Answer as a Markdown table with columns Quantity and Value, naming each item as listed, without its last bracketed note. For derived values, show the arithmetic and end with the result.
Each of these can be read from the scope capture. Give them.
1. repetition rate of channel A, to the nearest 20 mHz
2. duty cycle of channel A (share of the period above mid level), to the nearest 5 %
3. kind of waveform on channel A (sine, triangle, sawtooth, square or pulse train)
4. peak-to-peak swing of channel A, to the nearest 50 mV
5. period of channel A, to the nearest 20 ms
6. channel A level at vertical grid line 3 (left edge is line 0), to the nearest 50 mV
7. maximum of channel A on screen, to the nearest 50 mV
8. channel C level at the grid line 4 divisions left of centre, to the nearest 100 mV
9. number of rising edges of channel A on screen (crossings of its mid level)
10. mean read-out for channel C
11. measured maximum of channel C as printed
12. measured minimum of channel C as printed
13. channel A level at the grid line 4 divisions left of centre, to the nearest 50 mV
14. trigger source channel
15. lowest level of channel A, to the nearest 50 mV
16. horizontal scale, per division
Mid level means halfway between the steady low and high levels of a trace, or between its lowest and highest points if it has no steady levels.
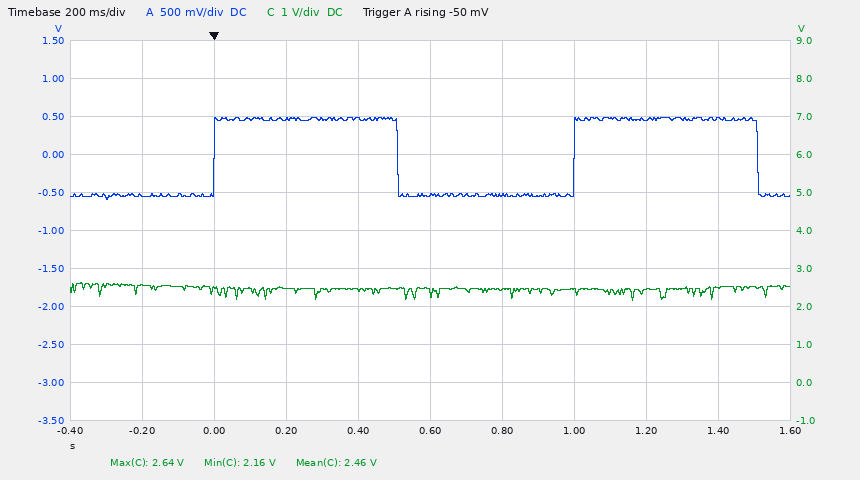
| Quantity | Value |
|---|---|
| repetition rate of channel A, to the nearest 20 mHz | 1 / 1.00 s ≈ 1.00 Hz |
| duty cycle of channel A (share of the period above mid level), to the nearest 5 % | 50 % |
| kind of waveform on channel A | square |
| peak-to-peak swing of channel A, to the nearest 50 mV | 500 mV − (-600 mV) = 1.10 V |
| period of channel A, to the nearest 20 ms | 1.00 s |
| channel A level at vertical grid line 3 (left edge is line 0), to the nearest 50 mV | 450 mV |
| maximum of channel A on screen, to the nearest 50 mV | 500 mV |
| channel C level at the grid line 4 divisions left of centre, to the nearest 100 mV | 2.6 V |
| number of rising edges of channel A on screen | 2 |
| mean read-out for channel C | 2.46 V |
| measured maximum of channel C as printed | 2.64 V |
| measured minimum of channel C as printed | 2.16 V |
| channel A level at the grid line 4 divisions left of centre, to the nearest 50 mV | -550 mV |
| trigger source channel | channel A |
| lowest level of channel A, to the nearest 50 mV | -600 mV |
| horizontal scale, per division | 200 ms |
